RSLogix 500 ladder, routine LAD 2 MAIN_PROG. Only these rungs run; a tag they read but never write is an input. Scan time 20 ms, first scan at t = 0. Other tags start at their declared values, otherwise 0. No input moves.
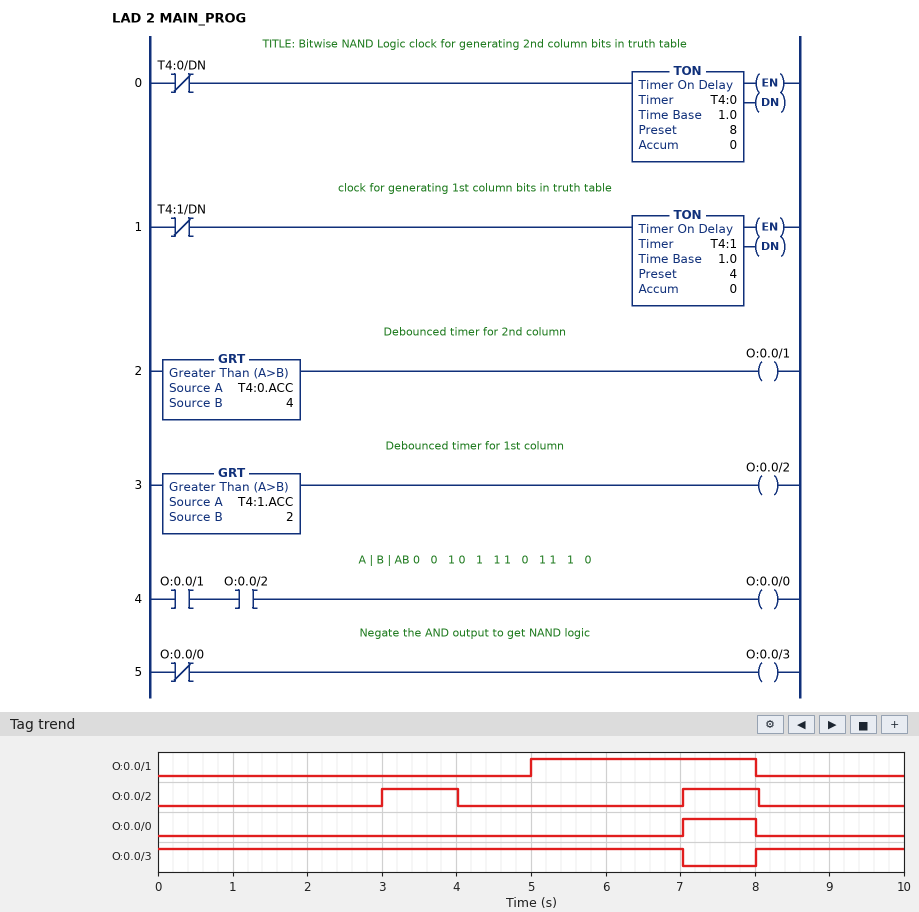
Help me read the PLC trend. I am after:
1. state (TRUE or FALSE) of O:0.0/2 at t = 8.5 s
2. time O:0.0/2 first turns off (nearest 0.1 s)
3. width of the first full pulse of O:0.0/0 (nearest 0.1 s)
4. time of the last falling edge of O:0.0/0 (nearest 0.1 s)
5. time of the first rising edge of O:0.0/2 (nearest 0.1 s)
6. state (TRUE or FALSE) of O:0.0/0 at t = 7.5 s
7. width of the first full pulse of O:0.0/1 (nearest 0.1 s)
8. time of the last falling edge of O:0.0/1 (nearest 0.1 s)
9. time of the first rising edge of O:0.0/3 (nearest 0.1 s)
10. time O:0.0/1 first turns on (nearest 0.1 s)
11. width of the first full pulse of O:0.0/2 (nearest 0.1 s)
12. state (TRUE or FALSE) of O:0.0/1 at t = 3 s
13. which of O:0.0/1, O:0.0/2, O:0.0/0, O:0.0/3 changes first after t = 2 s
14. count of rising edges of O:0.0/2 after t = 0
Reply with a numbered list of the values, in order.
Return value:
1. FALSE
2. 4.0 s
3. 1.0 s
4. 8.0 s
5. 3.0 s
6. TRUE
7. 3.0 s
8. 8.0 s
9. 8.0 s
10. 5.0 s
11. 1.0 s
12. FALSE
13. O:0.0/2
14. 2
